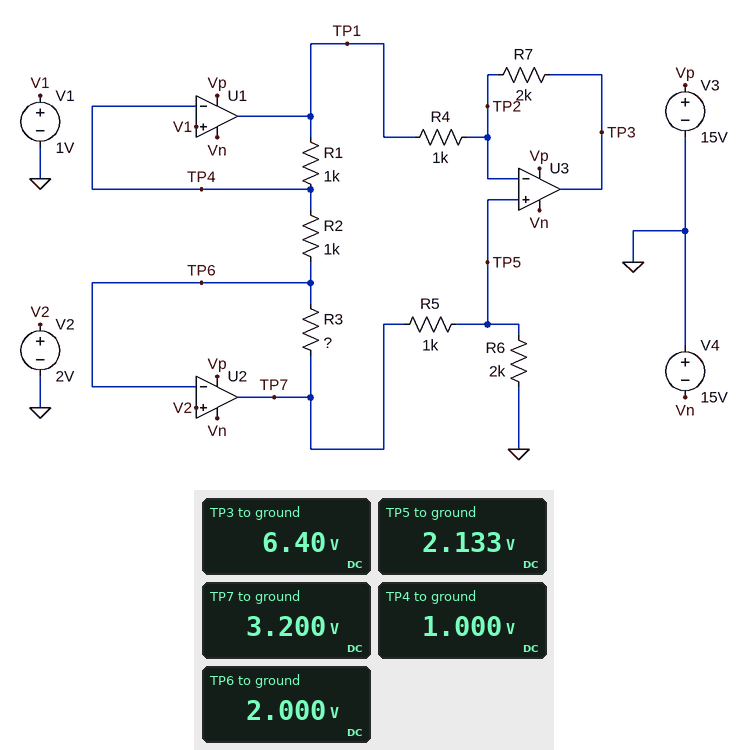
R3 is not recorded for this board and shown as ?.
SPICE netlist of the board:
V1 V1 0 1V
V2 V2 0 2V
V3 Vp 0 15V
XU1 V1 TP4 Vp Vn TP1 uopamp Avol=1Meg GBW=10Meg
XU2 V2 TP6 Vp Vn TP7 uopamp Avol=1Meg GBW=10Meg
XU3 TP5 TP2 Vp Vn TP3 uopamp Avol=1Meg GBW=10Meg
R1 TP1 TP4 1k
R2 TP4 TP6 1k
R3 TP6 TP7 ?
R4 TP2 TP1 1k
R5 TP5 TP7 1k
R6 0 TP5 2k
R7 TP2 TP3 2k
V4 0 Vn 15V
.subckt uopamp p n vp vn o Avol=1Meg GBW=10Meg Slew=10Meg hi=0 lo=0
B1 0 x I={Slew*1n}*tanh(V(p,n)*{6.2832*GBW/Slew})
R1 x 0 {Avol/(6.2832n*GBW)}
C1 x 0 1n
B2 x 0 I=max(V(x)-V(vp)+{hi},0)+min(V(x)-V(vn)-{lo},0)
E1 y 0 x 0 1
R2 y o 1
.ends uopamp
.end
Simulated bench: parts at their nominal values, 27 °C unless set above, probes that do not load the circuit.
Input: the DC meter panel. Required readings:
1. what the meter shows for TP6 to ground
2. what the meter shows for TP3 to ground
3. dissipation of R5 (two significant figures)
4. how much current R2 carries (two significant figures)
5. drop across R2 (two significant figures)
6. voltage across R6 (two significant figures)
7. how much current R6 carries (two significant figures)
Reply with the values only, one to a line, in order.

2.000 V
6.40 V
1.1 mW
1.0 mA
1.0 V
2.1 V
1.1 mA
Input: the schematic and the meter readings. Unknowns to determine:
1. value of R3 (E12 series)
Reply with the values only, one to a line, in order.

1.2 kΩ
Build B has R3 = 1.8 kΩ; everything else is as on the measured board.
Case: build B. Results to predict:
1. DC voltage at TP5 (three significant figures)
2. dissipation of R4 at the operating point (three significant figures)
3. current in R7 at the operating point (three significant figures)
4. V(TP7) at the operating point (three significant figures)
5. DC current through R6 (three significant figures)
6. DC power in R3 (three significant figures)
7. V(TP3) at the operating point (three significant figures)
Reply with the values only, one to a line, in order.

2.53 V
6.42 mW
2.53 mA
3.80 V
1.27 mA
1.80 mW
7.60 V
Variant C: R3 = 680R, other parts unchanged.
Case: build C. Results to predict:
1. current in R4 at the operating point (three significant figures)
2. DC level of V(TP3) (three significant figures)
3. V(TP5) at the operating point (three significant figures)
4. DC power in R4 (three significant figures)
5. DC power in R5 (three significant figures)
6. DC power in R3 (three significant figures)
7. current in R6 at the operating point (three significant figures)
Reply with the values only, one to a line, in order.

1.79 mA
5.36 V
1.79 V
3.19 mW
798 µW
680 µW
893 µA
